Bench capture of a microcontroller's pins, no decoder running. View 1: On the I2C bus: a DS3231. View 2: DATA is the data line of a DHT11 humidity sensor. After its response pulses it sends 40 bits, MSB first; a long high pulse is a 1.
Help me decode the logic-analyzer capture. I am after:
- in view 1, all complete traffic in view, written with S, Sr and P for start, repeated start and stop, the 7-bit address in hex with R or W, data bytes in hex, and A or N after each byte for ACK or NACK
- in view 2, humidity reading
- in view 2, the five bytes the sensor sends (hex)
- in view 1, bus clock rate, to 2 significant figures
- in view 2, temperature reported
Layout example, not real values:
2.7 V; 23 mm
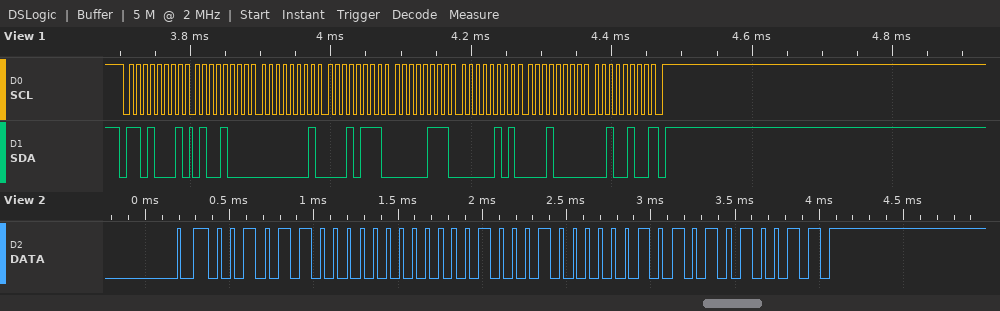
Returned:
S 68R A 48 A 01 A 17 A 07 A 05 A 10 A 24 N P; 44 %; 2C 00 22 05 53; 100 kHz; 34.5 °C
